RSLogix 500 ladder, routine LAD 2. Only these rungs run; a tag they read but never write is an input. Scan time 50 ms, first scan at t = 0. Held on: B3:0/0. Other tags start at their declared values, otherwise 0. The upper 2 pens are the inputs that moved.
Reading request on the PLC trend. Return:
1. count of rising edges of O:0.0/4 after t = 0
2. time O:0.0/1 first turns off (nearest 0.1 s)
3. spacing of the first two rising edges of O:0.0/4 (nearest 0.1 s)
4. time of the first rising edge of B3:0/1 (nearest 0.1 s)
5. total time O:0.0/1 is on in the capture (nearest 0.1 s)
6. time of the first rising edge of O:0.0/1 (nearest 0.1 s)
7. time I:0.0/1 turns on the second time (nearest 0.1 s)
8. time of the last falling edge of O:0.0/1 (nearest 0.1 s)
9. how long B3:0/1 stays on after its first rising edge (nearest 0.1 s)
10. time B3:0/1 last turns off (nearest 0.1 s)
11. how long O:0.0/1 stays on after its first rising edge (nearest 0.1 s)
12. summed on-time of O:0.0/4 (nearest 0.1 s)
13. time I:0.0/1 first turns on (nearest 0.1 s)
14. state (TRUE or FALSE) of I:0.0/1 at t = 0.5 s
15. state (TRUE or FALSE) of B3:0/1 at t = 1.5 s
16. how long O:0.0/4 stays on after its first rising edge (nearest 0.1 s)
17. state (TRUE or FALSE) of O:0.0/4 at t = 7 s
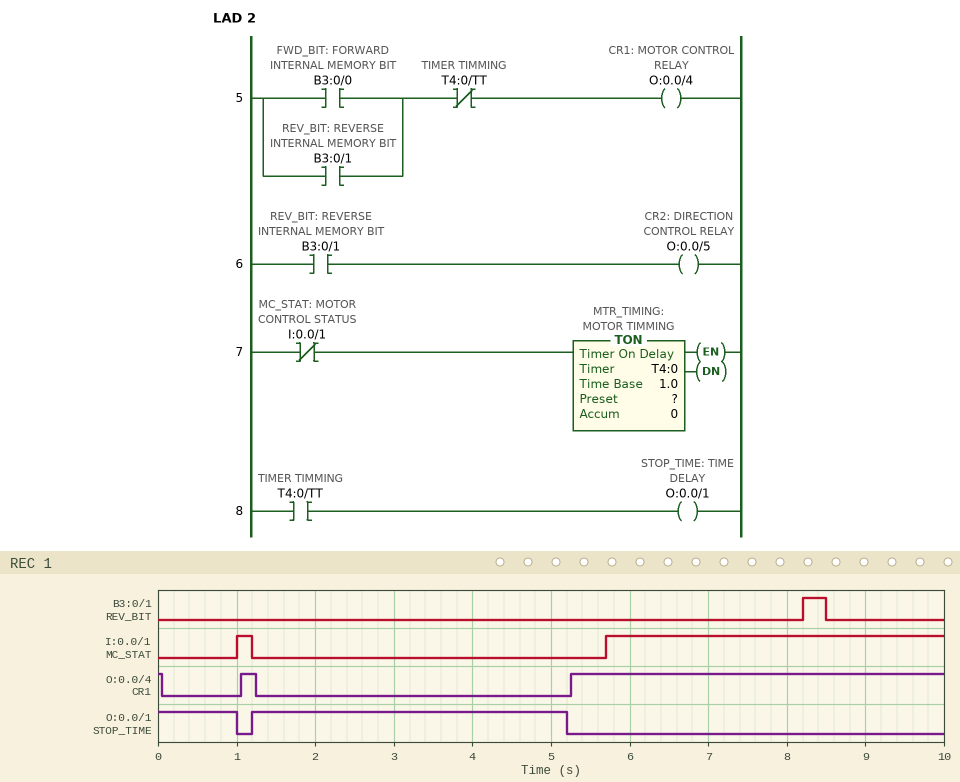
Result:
2
1.0 s
4.2 s
8.2 s
5.0 s
1.2 s
5.7 s
5.2 s
0.3 s
8.5 s
4.0 s
5.0 s
1.0 s
FALSE
FALSE
0.2 s
TRUE
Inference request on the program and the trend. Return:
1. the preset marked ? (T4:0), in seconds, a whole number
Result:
4 s
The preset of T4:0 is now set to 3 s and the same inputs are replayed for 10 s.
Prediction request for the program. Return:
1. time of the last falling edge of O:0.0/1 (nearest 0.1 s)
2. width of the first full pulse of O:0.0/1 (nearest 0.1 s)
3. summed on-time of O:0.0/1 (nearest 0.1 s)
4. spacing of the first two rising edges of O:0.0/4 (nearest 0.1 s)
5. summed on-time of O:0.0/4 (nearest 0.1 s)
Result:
4.2 s
3.0 s
4.0 s
3.2 s
6.0 s
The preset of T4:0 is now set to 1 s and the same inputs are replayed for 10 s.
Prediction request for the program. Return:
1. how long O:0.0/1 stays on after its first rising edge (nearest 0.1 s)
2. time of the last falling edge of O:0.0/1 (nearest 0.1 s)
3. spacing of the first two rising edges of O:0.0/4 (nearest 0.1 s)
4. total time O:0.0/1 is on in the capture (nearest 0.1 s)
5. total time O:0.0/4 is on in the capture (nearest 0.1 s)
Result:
1.0 s
2.2 s
1.2 s
2.0 s
8.0 s
